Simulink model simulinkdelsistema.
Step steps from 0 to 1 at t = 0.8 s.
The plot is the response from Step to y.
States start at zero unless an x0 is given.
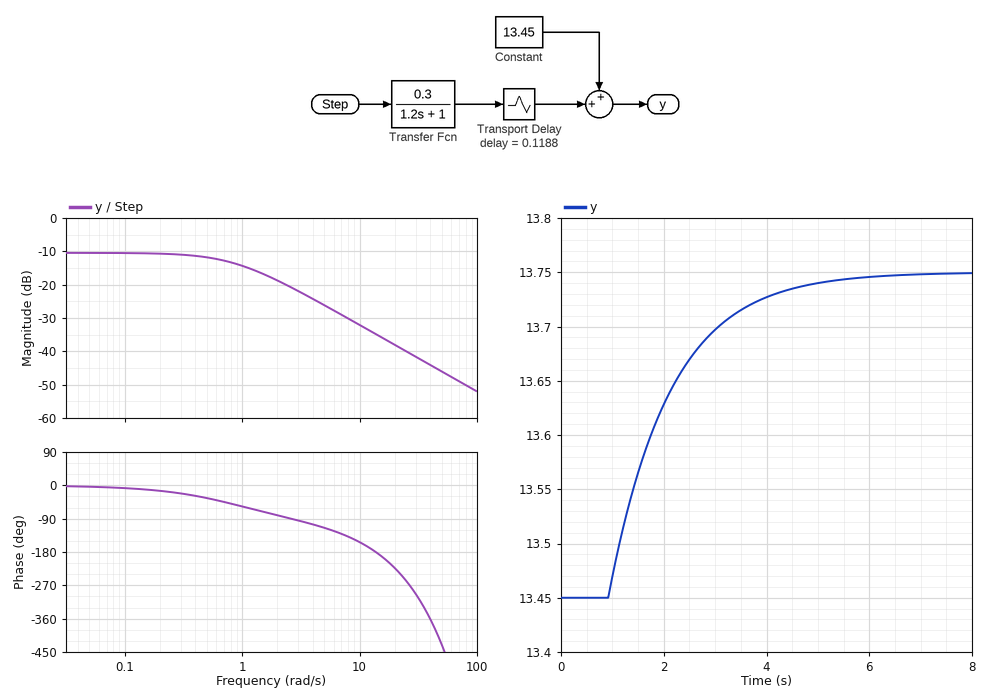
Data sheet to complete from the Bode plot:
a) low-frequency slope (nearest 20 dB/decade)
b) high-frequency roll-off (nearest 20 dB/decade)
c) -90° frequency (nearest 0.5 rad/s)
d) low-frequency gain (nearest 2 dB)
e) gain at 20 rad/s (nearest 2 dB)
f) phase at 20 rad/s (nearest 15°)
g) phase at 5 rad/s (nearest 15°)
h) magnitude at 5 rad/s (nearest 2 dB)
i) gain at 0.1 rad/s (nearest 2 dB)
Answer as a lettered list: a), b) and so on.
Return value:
a) 0 dB/decade
b) -20 dB/decade
c) 2.5 rad/s
d) -10 dB
e) -38 dB
f) -225°
g) -120°
h) -26 dB
i) -10 dB
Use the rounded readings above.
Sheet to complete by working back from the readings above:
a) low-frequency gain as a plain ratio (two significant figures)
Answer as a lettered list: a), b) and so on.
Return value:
a) 0.32
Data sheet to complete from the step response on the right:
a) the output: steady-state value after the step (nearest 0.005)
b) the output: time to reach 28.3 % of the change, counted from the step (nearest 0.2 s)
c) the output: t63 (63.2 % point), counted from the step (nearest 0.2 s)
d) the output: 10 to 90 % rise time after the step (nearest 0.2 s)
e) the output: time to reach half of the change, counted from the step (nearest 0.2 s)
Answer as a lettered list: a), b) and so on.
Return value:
a) 13.750
b) 0.6 s
c) 1.4 s
d) 2.6 s
e) 1.0 s
